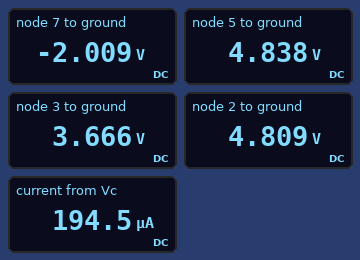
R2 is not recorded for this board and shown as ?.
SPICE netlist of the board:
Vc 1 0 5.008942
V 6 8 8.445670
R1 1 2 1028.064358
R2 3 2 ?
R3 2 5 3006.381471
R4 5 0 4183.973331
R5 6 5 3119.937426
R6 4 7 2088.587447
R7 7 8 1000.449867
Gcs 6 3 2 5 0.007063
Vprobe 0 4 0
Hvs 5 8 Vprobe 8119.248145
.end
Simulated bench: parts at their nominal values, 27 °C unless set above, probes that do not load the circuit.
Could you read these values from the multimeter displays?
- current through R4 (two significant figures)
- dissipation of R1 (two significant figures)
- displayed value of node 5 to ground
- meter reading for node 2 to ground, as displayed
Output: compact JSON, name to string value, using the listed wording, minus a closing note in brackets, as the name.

{"current through R4": "1.2 mA", "dissipation of R1": "39 µW", "displayed value of node 5 to ground": "4.838 V", "meter reading for node 2 to ground, as displayed": "4.809 V"}
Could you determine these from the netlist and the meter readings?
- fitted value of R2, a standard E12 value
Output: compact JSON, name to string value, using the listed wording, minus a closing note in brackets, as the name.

{"fitted value of R2, a standard E12 value": "5.6 kΩ"}
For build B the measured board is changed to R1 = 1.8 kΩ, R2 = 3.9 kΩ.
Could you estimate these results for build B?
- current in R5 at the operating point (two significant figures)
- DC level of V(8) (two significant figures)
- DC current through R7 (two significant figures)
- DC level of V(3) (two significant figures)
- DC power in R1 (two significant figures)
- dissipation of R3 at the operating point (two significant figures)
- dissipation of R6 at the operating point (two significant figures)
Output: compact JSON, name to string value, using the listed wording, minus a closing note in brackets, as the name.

{"current in R5 at the operating point": "280 µA", "DC level of V(8)": "-2.9 V", "DC current through R7": "930 µA", "DC level of V(3)": "3.9 V", "DC power in R1": "64 µW", "dissipation of R3 at the operating point": "260 nW", "dissipation of R6 at the operating point": "1.8 mW"}
